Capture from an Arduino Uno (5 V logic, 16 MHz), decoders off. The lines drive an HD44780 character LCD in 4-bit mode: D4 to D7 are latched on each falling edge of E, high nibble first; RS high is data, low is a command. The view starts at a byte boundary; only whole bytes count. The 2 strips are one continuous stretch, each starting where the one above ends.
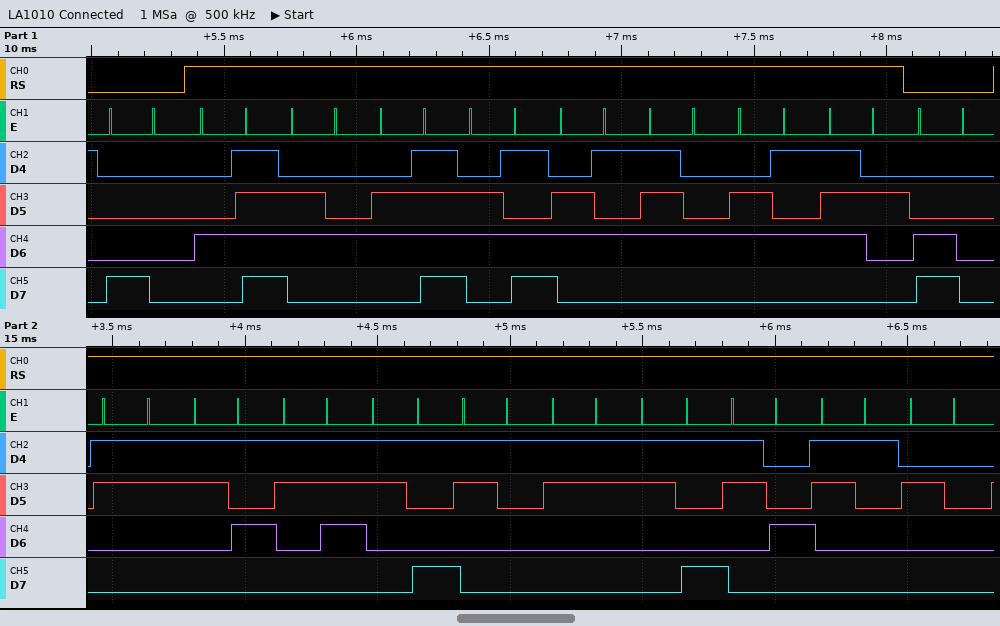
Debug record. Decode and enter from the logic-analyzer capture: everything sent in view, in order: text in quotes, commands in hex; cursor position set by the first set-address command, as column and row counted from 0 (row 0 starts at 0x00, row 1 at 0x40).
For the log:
0x80 "Odometer" 0xC0 "357913941 "
column 0, row 0
